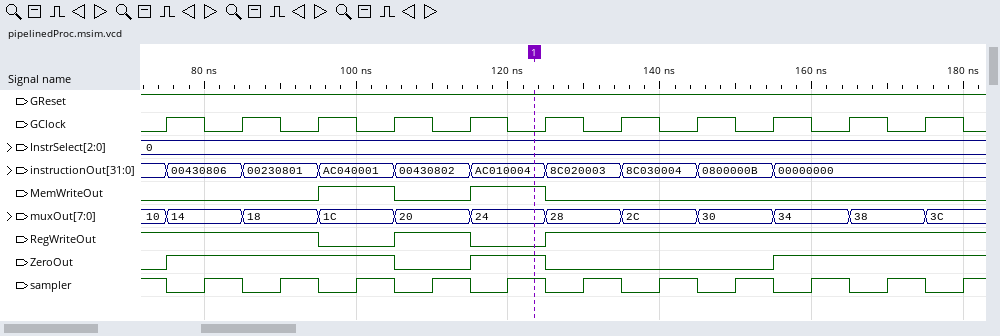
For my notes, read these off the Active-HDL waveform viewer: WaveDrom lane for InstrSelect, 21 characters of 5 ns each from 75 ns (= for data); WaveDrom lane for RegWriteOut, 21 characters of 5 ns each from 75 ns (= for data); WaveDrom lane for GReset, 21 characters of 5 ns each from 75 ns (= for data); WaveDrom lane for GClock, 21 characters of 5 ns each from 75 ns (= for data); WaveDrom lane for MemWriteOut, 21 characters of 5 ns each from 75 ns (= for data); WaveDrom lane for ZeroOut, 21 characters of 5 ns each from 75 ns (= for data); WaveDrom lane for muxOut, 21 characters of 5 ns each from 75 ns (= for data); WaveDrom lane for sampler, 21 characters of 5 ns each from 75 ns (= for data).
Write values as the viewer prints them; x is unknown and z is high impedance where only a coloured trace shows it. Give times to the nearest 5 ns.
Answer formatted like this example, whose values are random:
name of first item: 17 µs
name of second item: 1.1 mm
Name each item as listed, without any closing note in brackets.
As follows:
WaveDrom lane for InstrSelect, 21 characters of 5 ns each from 75 ns: {name: 'InstrSelect', wave: '=....................', data: '0'}
WaveDrom lane for RegWriteOut, 21 characters of 5 ns each from 75 ns: {name: 'RegWriteOut', wave: '1...0.1.0.1..........'}
WaveDrom lane for GReset, 21 characters of 5 ns each from 75 ns: {name: 'GReset', wave: '1....................'}
WaveDrom lane for GClock, 21 characters of 5 ns each from 75 ns: {name: 'GClock', wave: '101010101010101010101'}
WaveDrom lane for MemWriteOut, 21 characters of 5 ns each from 75 ns: {name: 'MemWriteOut', wave: '0...1.0.1.0..........'}
WaveDrom lane for ZeroOut, 21 characters of 5 ns each from 75 ns: {name: 'ZeroOut', wave: '1.....0.1.0.....1....'}
WaveDrom lane for muxOut, 21 characters of 5 ns each from 75 ns: {name: 'muxOut', wave: '=.=.=.=.=.=.=.=.=.=.=', data: '14 18 1C 20 24 28 2C 30 34 38 3C'}
WaveDrom lane for sampler, 21 characters of 5 ns each from 75 ns: {name: 'sampler', wave: '010101010101010101010'}
